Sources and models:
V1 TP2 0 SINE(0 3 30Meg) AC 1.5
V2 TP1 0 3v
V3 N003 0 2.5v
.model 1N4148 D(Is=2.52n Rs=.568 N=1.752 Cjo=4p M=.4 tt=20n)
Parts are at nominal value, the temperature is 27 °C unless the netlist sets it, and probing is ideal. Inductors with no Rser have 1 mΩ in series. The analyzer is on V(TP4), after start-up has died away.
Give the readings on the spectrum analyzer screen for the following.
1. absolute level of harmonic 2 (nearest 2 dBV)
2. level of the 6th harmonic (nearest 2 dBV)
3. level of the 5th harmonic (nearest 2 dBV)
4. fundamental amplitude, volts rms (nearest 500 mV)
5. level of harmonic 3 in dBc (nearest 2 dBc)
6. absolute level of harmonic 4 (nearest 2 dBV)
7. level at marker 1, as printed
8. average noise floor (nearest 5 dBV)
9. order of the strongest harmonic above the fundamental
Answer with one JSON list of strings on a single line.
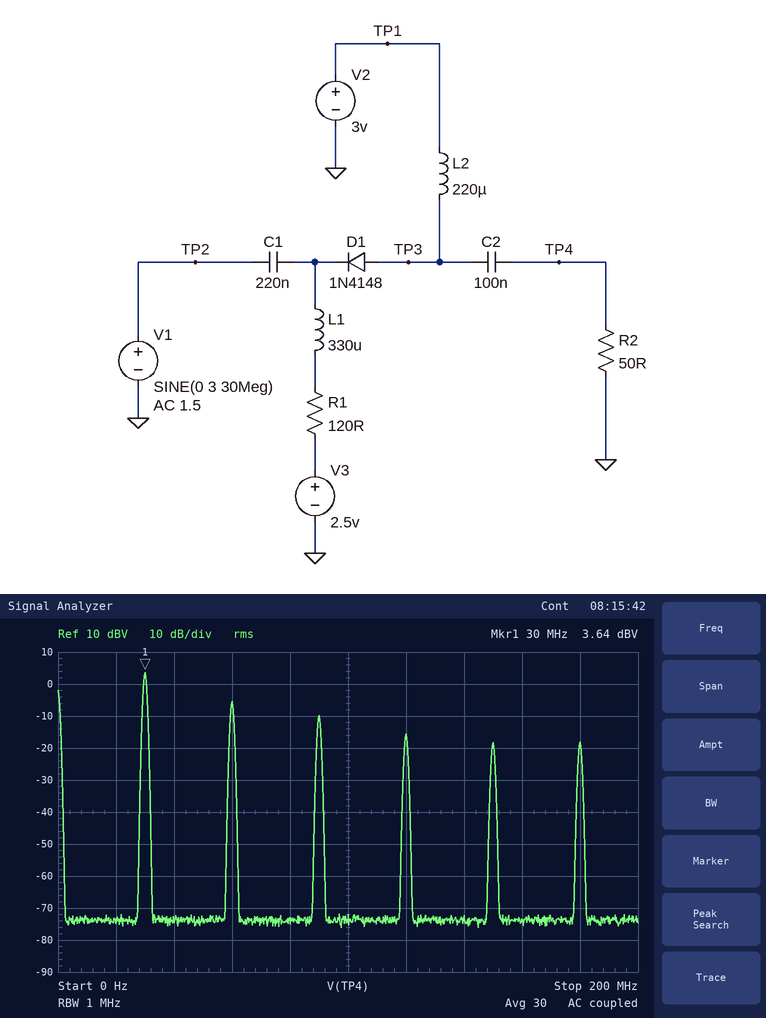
["-6 dBV", "-18 dBV", "-18 dBV", "1.5 V", "-14 dBc", "-16 dBV", "3.64 dBV", "-75 dBV", "2"]
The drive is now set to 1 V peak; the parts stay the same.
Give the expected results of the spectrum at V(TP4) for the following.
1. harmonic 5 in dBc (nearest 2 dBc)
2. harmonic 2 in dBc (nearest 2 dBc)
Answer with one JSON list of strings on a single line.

["-20 dBc", "-8 dBc"]
